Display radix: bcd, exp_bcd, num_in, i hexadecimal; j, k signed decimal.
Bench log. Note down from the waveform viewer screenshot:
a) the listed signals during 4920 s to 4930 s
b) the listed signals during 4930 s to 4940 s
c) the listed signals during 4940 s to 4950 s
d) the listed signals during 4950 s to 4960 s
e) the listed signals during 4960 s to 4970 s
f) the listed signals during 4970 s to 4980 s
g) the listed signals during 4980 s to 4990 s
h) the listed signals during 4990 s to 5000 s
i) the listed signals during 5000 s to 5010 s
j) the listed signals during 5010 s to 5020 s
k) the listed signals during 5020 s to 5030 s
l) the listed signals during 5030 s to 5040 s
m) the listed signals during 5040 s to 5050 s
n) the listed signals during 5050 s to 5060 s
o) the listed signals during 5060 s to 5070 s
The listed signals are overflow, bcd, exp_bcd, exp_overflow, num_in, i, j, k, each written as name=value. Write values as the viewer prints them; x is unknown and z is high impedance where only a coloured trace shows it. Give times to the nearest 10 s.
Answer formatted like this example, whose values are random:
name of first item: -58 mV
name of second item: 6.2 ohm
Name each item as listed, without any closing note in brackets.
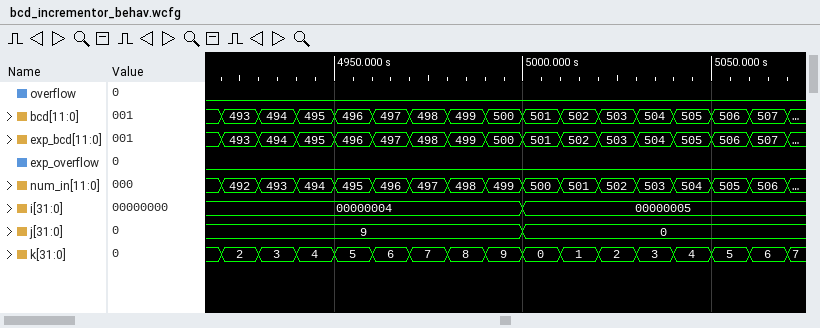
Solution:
the listed signals during 4920 s to 4930 s: overflow=0, bcd=493, exp_bcd=493, exp_overflow=0, num_in=492, i=00000004, j=9, k=2
the listed signals during 4930 s to 4940 s: overflow=0, bcd=494, exp_bcd=494, exp_overflow=0, num_in=493, i=00000004, j=9, k=3
the listed signals during 4940 s to 4950 s: overflow=0, bcd=495, exp_bcd=495, exp_overflow=0, num_in=494, i=00000004, j=9, k=4
the listed signals during 4950 s to 4960 s: overflow=0, bcd=496, exp_bcd=496, exp_overflow=0, num_in=495, i=00000004, j=9, k=5
the listed signals during 4960 s to 4970 s: overflow=0, bcd=497, exp_bcd=497, exp_overflow=0, num_in=496, i=00000004, j=9, k=6
the listed signals during 4970 s to 4980 s: overflow=0, bcd=498, exp_bcd=498, exp_overflow=0, num_in=497, i=00000004, j=9, k=7
the listed signals during 4980 s to 4990 s: overflow=0, bcd=499, exp_bcd=499, exp_overflow=0, num_in=498, i=00000004, j=9, k=8
the listed signals during 4990 s to 5000 s: overflow=0, bcd=500, exp_bcd=500, exp_overflow=0, num_in=499, i=00000004, j=9, k=9
the listed signals during 5000 s to 5010 s: overflow=0, bcd=501, exp_bcd=501, exp_overflow=0, num_in=500, i=00000005, j=0, k=0
the listed signals during 5010 s to 5020 s: overflow=0, bcd=502, exp_bcd=502, exp_overflow=0, num_in=501, i=00000005, j=0, k=1
the listed signals during 5020 s to 5030 s: overflow=0, bcd=503, exp_bcd=503, exp_overflow=0, num_in=502, i=00000005, j=0, k=2
the listed signals during 5030 s to 5040 s: overflow=0, bcd=504, exp_bcd=504, exp_overflow=0, num_in=503, i=00000005, j=0, k=3
the listed signals during 5040 s to 5050 s: overflow=0, bcd=505, exp_bcd=505, exp_overflow=0, num_in=504, i=00000005, j=0, k=4
the listed signals during 5050 s to 5060 s: overflow=0, bcd=506, exp_bcd=506, exp_overflow=0, num_in=505, i=00000005, j=0, k=5
the listed signals during 5060 s to 5070 s: overflow=0, bcd=507, exp_bcd=507, exp_overflow=0, num_in=506, i=00000005, j=0, k=6
